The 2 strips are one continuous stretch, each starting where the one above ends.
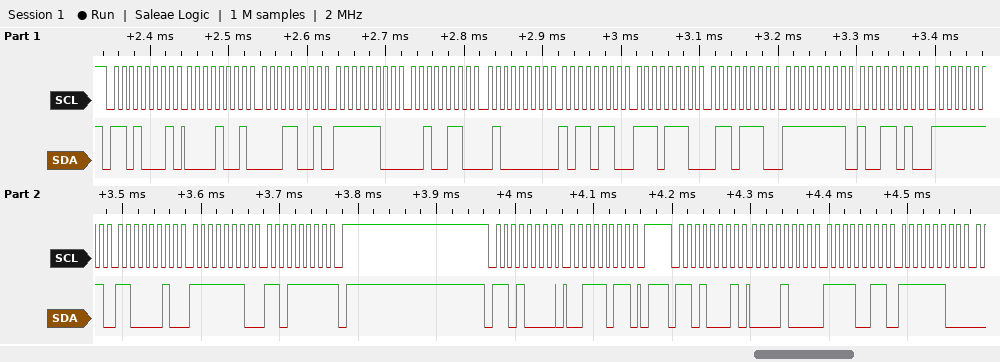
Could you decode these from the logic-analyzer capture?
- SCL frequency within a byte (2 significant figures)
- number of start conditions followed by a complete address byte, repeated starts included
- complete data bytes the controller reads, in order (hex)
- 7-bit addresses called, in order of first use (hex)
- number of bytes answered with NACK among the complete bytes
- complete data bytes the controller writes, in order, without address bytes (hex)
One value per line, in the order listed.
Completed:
100 kHz
3
09 19 FC 26 40 B6 EE 6E FF 9A FF C2 FE DF 08 F3 FC
0x68
1
3B
